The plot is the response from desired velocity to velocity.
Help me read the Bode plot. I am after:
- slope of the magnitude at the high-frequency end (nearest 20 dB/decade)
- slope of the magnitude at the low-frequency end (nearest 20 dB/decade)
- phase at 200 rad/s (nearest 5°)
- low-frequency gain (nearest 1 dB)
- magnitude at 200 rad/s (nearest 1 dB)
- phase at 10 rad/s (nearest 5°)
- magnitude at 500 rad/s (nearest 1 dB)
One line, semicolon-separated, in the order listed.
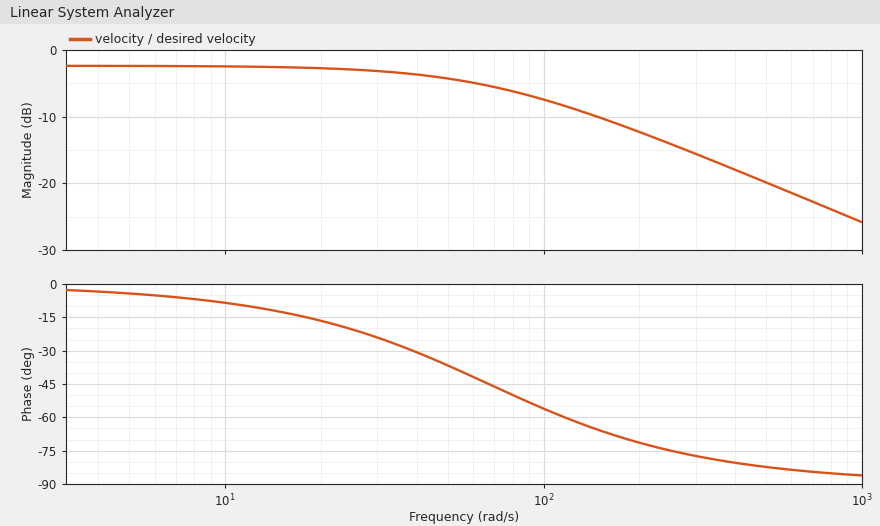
-20 dB/decade; 0 dB/decade; -70°; -2 dB; -12 dB; -10°; -20 dB
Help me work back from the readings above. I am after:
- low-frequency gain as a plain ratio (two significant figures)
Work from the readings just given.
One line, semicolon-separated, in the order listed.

0.79
